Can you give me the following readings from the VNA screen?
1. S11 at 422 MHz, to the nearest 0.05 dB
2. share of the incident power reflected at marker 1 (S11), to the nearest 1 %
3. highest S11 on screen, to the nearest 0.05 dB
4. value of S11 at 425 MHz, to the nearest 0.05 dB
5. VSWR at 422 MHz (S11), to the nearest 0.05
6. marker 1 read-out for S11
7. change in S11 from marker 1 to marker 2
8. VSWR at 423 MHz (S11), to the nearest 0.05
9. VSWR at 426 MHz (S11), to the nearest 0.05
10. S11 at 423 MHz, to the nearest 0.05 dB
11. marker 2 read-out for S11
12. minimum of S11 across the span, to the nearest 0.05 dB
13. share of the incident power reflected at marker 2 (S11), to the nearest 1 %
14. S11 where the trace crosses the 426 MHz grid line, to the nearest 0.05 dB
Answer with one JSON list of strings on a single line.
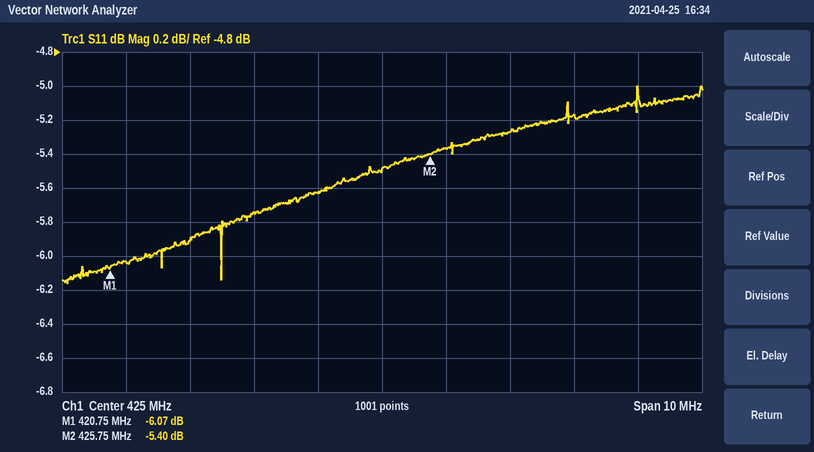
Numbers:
["-5.90 dB", "25 %", "-5.00 dB", "-5.50 dB", "3.05", "-6.07 dB", "0.67 dB", "3.15", "3.35", "-5.75 dB", "-5.40 dB", "-6.15 dB", "29 %", "-5.35 dB"]
